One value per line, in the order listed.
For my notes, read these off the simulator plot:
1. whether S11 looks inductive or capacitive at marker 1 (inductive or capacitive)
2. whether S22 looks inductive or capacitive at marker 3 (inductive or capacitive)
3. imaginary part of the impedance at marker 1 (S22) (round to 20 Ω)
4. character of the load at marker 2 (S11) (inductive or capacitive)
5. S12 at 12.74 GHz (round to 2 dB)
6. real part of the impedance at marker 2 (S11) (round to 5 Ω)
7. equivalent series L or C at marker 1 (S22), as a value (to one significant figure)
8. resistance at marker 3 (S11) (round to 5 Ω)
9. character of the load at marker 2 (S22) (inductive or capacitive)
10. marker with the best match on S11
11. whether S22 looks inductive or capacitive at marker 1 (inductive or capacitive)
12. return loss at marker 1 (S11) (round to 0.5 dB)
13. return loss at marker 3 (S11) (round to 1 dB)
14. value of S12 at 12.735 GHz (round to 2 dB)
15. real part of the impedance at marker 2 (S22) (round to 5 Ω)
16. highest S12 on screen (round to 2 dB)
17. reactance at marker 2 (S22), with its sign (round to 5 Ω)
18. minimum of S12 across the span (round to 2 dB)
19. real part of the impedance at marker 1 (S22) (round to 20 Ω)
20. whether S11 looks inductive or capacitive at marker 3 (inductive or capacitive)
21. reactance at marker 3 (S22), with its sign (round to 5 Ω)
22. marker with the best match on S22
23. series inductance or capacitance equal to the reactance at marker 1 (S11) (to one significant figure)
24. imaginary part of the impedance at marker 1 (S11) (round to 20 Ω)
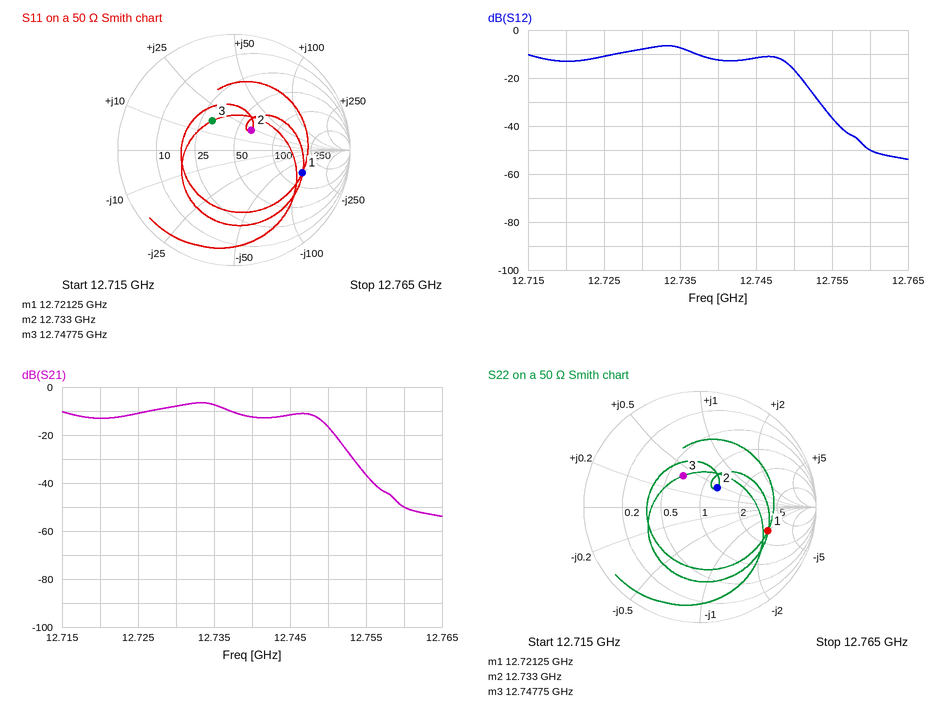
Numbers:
capacitive
inductive
-100 Ω
inductive
-12 dB
65 Ω
100 fF
30 Ω
inductive
marker 2
capacitive
4.0 dB
10 dB
-8 dB
65 Ω
-6 dB
+20 Ω
-54 dB
140 Ω
inductive
+20 Ω
marker 2
100 fF
-100 Ω
